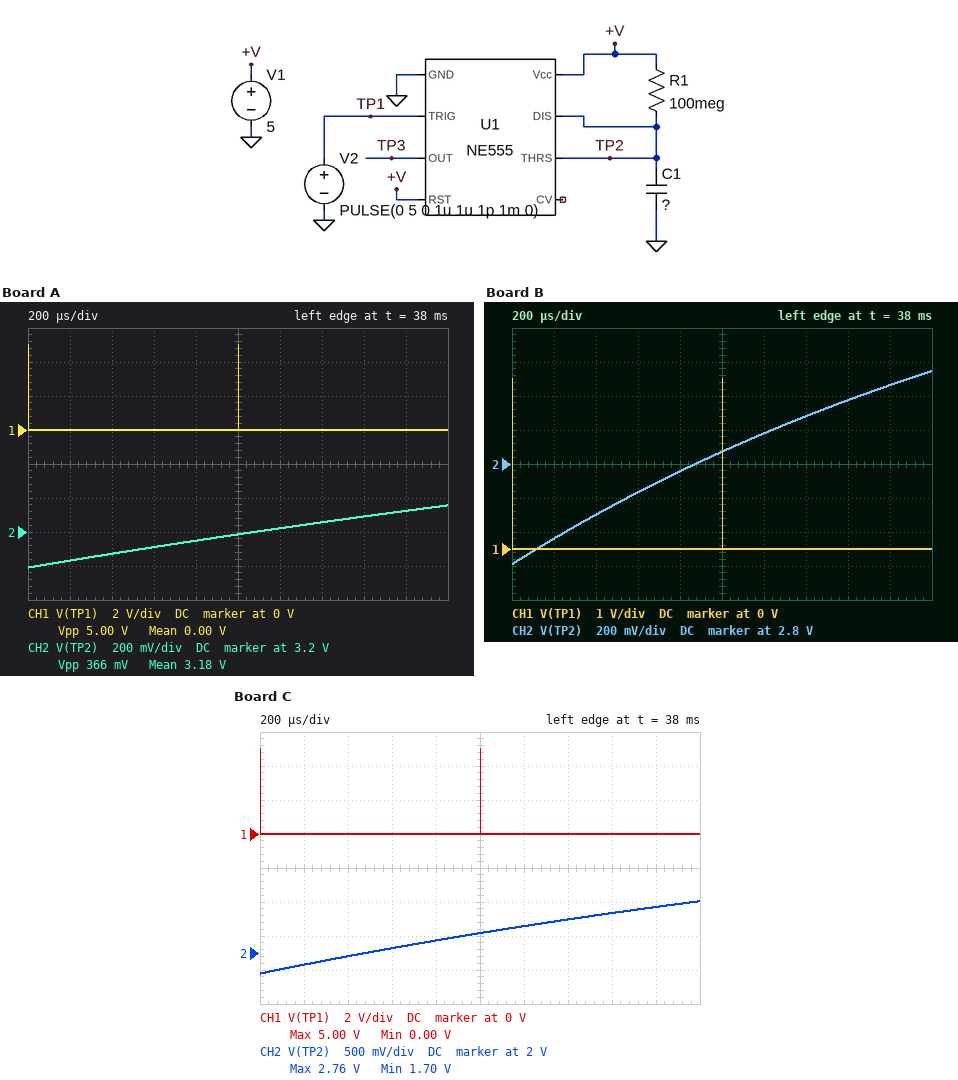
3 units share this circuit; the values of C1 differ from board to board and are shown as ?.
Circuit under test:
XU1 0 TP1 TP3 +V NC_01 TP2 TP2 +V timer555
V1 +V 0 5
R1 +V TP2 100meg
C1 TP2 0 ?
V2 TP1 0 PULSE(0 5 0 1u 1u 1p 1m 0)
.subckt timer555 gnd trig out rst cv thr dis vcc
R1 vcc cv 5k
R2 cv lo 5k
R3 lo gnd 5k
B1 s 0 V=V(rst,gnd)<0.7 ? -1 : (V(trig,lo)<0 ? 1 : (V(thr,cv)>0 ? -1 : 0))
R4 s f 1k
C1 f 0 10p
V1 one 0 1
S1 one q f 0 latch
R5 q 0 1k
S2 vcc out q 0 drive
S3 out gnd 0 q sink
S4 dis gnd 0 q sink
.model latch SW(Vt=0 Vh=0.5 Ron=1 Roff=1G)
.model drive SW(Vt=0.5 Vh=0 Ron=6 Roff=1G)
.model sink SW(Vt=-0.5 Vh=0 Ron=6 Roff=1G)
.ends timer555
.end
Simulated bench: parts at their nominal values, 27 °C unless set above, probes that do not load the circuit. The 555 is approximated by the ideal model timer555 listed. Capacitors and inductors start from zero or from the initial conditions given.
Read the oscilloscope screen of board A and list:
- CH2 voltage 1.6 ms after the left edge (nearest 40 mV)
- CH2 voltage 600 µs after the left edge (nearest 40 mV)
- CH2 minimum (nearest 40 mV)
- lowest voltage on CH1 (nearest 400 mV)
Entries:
3.28 V
3.12 V
3.00 V
0 V
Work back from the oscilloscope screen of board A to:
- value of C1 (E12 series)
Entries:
82 pF
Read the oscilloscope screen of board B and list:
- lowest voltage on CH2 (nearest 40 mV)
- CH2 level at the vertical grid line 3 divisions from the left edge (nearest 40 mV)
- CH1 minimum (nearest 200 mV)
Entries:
2.20 V
2.64 V
0 V
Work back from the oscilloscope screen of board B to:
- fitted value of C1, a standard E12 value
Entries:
33 pF
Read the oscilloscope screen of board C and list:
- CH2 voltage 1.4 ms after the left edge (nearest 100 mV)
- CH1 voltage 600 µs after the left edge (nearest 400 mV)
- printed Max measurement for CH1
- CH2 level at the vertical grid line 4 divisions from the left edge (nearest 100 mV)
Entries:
2.5 V
0 V
5.00 V
2.2 V
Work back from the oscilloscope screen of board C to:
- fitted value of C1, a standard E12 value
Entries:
47 pF
